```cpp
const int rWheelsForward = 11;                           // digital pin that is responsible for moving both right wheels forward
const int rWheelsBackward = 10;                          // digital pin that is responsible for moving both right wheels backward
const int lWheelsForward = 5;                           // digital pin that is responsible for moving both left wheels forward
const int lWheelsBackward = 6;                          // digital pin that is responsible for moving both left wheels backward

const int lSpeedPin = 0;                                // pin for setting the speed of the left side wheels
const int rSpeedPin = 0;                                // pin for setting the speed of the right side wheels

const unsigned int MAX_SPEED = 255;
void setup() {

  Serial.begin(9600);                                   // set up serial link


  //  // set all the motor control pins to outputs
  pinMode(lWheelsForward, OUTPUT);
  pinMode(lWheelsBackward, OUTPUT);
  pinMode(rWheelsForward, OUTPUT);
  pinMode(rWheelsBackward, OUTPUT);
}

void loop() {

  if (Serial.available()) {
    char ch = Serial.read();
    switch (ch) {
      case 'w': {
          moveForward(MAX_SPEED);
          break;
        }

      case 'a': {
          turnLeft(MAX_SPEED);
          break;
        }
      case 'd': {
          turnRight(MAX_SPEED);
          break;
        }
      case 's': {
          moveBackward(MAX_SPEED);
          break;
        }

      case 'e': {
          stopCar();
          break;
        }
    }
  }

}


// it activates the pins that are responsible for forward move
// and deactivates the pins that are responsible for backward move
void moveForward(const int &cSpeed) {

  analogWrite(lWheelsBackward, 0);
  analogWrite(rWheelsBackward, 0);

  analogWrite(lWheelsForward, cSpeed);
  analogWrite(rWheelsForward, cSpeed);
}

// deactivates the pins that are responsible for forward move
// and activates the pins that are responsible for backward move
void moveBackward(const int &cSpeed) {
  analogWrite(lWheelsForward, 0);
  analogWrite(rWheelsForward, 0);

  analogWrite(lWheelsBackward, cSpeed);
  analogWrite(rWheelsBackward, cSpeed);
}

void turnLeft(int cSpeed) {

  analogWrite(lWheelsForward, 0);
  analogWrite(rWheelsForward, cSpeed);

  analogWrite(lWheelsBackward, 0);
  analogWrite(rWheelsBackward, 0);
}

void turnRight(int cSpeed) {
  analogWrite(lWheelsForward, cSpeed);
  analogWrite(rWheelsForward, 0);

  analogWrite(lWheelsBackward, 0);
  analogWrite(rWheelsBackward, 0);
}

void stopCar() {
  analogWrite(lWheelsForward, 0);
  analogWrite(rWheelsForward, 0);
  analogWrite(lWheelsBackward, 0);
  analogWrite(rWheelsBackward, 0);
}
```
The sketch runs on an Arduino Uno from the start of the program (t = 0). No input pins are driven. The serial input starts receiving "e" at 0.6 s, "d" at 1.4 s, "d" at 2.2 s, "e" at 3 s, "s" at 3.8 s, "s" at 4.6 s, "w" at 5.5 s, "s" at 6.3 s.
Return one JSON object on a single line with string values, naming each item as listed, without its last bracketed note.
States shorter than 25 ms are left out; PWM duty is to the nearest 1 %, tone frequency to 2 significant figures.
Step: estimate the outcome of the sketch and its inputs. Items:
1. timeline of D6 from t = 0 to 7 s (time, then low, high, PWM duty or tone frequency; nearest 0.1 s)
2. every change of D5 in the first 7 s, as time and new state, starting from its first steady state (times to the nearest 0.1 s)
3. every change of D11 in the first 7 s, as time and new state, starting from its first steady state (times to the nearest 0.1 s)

{"timeline of D6 from t = 0 to 7 s": "0 s low; 3.8 s high; 5.5 s low; 6.3 s high", "every change of D5 in the first 7 s, as time and new state, starting from its first steady state": "0 s low; 1.4 s high; 3 s low; 5.5 s high; 6.3 s low", "every change of D11 in the first 7 s, as time and new state, starting from its first steady state": "0 s low; 5.5 s high; 6.3 s low"}
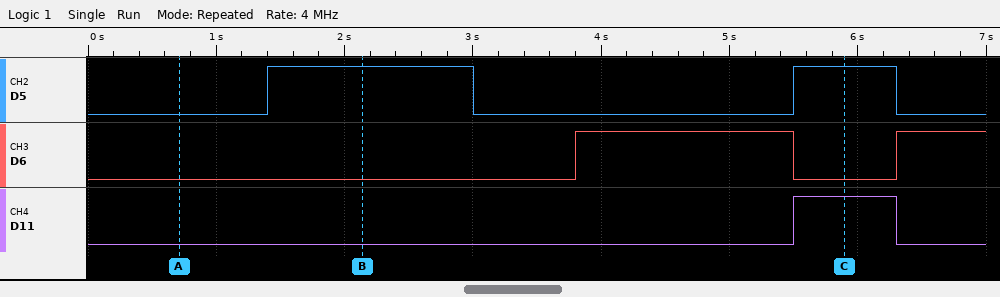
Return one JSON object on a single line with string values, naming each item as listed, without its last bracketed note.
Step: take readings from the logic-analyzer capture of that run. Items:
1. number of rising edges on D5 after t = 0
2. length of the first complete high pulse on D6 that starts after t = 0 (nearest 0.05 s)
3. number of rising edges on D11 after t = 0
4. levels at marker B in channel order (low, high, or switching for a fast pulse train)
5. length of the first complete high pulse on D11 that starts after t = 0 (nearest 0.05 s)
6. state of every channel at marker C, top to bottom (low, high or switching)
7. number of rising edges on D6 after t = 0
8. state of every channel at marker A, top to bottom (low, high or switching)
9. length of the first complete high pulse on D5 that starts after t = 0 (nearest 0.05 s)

{"number of rising edges on D5 after t = 0": "2", "length of the first complete high pulse on D6 that starts after t = 0": "1.70 s", "number of rising edges on D11 after t = 0": "1", "levels at marker B in channel order": "D5 high, D6 low, D11 low", "length of the first complete high pulse on D11 that starts after t = 0": "0.80 s", "state of every channel at marker C, top to bottom": "D5 high, D6 low, D11 high", "number of rising edges on D6 after t = 0": "2", "state of every channel at marker A, top to bottom": "D5 low, D6 low, D11 low", "length of the first complete high pulse on D5 that starts after t = 0": "1.60 s"}
